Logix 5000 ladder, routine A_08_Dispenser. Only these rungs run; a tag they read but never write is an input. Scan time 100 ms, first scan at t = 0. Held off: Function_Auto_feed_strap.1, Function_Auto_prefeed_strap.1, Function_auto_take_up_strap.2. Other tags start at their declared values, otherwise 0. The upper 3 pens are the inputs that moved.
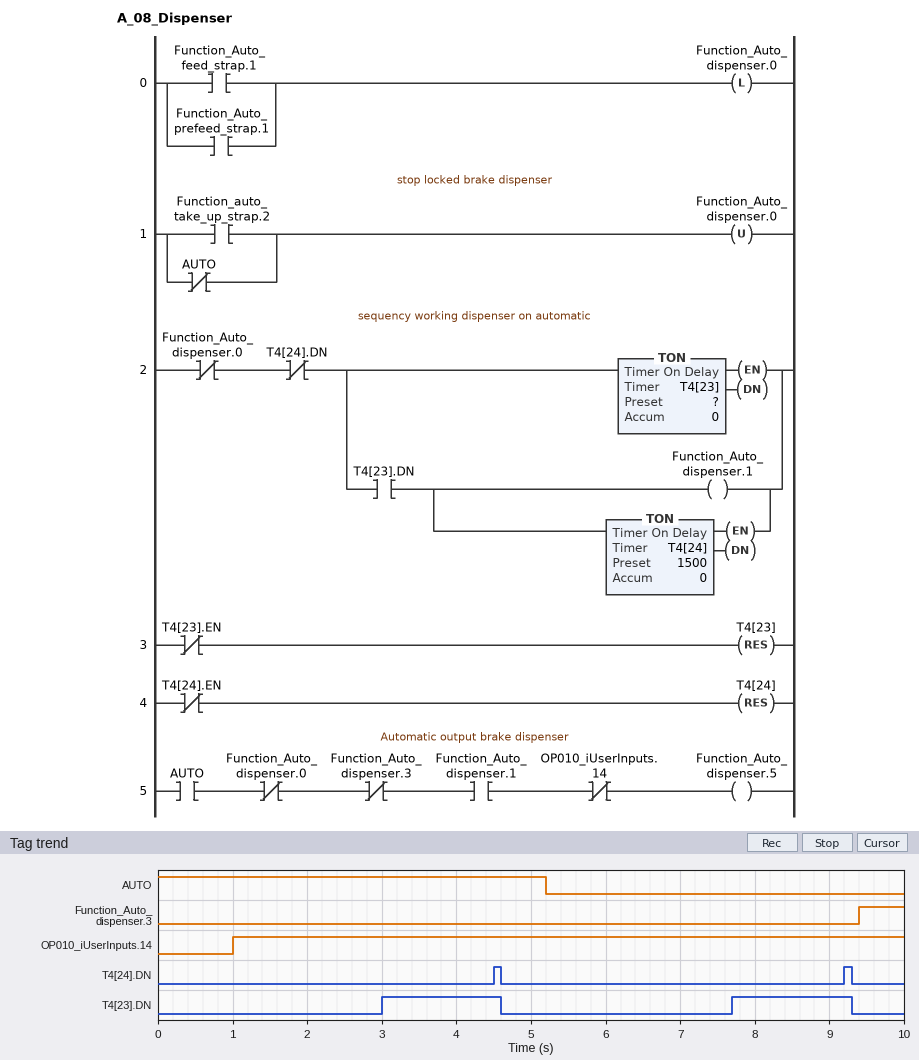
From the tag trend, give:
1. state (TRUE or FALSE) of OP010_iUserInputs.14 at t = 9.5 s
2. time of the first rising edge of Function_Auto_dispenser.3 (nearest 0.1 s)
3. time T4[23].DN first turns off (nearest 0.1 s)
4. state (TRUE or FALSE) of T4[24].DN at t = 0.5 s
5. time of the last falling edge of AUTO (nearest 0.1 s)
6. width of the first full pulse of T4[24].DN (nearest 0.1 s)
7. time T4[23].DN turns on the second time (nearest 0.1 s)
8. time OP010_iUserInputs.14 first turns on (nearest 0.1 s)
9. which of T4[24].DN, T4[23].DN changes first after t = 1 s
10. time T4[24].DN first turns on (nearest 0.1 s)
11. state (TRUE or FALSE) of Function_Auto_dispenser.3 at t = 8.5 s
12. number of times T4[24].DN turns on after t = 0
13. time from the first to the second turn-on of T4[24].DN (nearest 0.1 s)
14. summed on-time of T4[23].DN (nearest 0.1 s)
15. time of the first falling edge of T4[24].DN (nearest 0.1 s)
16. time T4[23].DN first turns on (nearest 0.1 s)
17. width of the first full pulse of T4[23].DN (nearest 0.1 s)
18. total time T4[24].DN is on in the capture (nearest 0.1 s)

TRUE
9.4 s
4.6 s
FALSE
5.2 s
0.1 s
7.7 s
1.0 s
T4[23].DN
4.5 s
FALSE
2
4.7 s
3.2 s
4.6 s
3.0 s
1.6 s
0.2 s
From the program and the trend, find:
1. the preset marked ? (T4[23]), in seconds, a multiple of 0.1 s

3.0 s
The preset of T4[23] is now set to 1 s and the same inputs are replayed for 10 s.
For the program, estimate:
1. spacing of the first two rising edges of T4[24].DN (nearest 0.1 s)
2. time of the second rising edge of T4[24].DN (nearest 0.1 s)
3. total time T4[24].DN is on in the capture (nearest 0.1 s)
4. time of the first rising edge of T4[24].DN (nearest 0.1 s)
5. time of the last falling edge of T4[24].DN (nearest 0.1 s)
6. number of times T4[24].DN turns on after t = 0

2.7 s
5.2 s
0.3 s
2.5 s
8.0 s
3
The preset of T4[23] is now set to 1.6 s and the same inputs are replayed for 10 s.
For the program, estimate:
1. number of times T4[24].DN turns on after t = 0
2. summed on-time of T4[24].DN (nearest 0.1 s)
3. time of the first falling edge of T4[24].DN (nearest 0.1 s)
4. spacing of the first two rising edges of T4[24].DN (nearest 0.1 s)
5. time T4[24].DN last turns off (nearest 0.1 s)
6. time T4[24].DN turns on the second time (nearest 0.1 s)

3
0.3 s
3.2 s
3.3 s
9.8 s
6.4 s
